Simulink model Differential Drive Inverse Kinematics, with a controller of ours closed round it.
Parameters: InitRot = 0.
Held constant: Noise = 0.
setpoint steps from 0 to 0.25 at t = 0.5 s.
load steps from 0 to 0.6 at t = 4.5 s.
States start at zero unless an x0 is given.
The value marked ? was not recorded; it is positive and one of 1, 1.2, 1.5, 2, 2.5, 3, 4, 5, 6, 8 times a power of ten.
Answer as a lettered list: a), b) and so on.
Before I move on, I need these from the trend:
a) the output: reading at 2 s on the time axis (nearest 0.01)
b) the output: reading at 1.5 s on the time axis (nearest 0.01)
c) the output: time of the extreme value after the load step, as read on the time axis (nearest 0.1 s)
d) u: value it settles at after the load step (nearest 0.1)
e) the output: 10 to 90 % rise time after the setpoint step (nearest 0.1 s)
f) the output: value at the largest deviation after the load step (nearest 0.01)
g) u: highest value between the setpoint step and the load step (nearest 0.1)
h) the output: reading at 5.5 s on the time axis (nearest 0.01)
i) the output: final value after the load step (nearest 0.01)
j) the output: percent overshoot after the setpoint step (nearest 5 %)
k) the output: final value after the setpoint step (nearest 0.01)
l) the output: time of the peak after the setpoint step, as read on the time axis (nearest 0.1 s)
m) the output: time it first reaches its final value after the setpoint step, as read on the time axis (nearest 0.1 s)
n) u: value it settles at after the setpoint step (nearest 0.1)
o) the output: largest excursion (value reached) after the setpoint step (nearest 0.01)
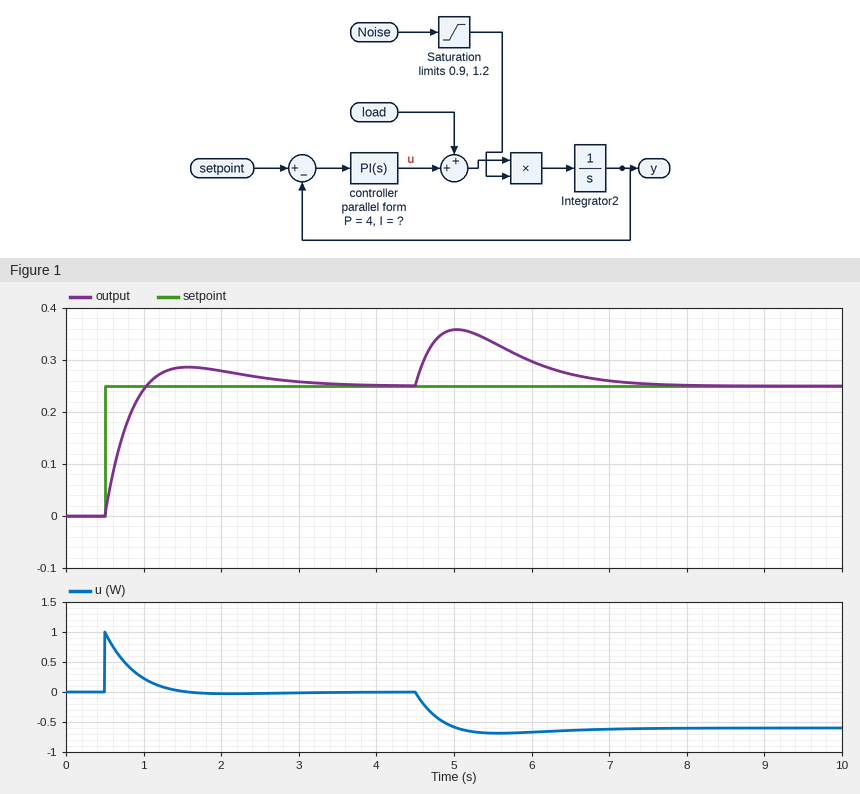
a) 0.28
b) 0.29
c) 5.0 s
d) -0.6
e) 0.4 s
f) 0.36
g) 1.0
h) 0.33
i) 0.25
j) 15 %
k) 0.25
l) 1.6 s
m) 1.0 s
n) 0.0
o) 0.29
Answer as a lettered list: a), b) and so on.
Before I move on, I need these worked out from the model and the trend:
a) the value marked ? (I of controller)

a) 4
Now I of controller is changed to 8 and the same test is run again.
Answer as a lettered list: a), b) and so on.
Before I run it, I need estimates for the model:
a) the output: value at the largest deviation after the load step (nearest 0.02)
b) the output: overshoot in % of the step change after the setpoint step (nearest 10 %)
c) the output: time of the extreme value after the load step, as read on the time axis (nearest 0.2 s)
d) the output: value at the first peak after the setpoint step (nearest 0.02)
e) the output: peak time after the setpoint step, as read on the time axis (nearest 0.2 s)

a) 0.34
b) 20 %
c) 5.0 s
d) 0.30
e) 1.4 s
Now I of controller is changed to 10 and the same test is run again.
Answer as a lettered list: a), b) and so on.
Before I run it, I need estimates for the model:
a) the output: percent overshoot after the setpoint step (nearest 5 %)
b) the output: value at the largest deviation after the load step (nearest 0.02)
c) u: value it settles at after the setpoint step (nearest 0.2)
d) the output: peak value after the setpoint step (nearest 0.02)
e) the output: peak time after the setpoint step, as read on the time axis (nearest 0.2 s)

a) 25 %
b) 0.34
c) 0.0
d) 0.32
e) 1.2 s
